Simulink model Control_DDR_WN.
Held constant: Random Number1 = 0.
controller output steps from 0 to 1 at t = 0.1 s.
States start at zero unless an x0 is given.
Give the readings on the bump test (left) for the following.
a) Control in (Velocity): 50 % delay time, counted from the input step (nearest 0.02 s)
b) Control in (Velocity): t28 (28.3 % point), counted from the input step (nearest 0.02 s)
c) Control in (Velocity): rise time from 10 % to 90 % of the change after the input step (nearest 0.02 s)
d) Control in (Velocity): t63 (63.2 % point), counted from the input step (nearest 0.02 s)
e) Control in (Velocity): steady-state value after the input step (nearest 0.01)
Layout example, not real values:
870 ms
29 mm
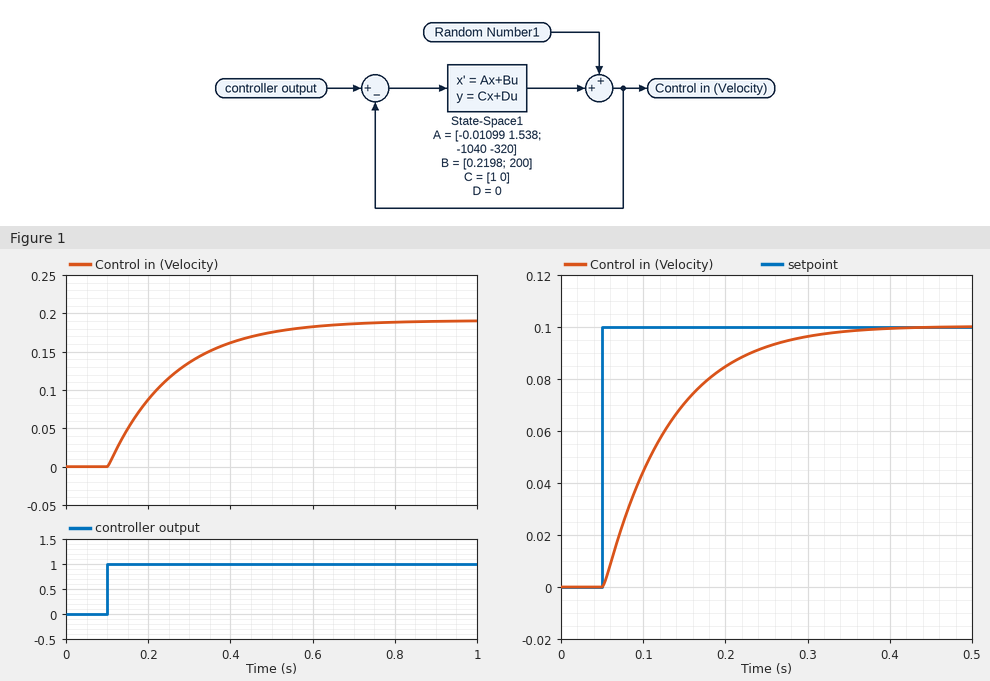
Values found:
0.12 s
0.06 s
0.34 s
0.16 s
0.19
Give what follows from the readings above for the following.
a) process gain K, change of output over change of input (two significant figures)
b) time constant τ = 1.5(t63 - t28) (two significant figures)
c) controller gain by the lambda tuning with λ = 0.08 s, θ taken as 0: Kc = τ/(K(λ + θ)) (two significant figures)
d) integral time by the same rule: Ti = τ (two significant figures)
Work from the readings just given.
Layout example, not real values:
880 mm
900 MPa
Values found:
0.19
0.15 s
9.9
0.15 s
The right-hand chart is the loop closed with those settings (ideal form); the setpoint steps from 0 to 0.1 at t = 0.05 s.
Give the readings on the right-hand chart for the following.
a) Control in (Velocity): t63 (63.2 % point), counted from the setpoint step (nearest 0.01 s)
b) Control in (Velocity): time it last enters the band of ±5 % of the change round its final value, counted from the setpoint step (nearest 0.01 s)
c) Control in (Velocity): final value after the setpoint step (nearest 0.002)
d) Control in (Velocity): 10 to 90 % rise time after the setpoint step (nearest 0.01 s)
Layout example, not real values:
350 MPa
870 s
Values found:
0.08 s
0.23 s
0.100
0.17 s
